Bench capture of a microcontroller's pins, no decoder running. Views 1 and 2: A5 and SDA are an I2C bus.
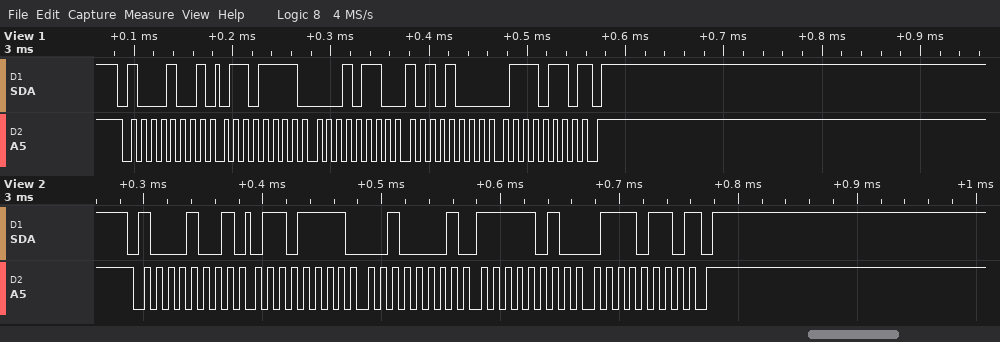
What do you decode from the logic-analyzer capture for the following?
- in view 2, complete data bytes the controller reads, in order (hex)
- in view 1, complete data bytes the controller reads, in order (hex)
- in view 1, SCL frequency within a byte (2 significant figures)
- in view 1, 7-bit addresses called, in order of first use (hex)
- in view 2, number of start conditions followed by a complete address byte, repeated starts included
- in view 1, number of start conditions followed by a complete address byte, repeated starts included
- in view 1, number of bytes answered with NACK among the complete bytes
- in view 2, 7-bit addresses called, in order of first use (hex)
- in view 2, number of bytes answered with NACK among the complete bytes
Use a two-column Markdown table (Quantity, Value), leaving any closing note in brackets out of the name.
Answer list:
| Quantity | Value |
|---|---|
| in view 2, complete data bytes the controller reads, in order | 6F 21 FA 76 |
| in view 1, complete data bytes the controller reads, in order | 6F 16 A8 76 |
| in view 1, SCL frequency within a byte | 100 kHz |
| in view 1, 7-bit addresses called, in order of first use | 0x44 |
| in view 2, number of start conditions followed by a complete address byte, repeated starts included | 1 |
| in view 1, number of start conditions followed by a complete address byte, repeated starts included | 1 |
| in view 1, number of bytes answered with NACK among the complete bytes | 1 |
| in view 2, 7-bit addresses called, in order of first use | 0x44 |
| in view 2, number of bytes answered with NACK among the complete bytes | 1 |
